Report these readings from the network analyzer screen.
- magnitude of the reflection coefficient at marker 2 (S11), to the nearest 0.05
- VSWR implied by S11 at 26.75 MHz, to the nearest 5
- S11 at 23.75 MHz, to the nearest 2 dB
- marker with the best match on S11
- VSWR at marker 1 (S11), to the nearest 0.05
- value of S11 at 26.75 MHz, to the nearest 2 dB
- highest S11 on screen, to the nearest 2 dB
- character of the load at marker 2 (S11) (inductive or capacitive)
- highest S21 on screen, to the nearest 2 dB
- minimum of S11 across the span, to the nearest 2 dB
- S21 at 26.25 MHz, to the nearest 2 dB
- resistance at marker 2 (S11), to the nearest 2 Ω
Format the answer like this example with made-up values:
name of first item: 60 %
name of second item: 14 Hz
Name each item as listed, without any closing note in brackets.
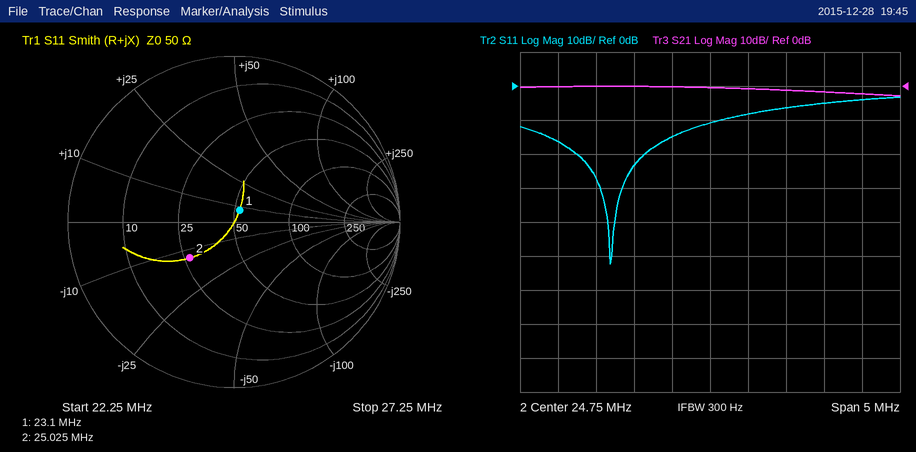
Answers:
magnitude of the reflection coefficient at marker 2 (S11), to the nearest 0.05: 0.35
VSWR implied by S11 at 26.75 MHz, to the nearest 5: 5
S11 at 23.75 MHz, to the nearest 2 dB: -24 dB
marker with the best match on S11: marker 1
VSWR at marker 1 (S11), to the nearest 0.05: 1.15
value of S11 at 26.75 MHz, to the nearest 2 dB: -4 dB
highest S11 on screen, to the nearest 2 dB: -4 dB
character of the load at marker 2 (S11): capacitive
highest S21 on screen, to the nearest 2 dB: 0 dB
minimum of S11 across the span, to the nearest 2 dB: -52 dB
S21 at 26.25 MHz, to the nearest 2 dB: -2 dB
resistance at marker 2 (S11), to the nearest 2 Ω: 26 Ω
